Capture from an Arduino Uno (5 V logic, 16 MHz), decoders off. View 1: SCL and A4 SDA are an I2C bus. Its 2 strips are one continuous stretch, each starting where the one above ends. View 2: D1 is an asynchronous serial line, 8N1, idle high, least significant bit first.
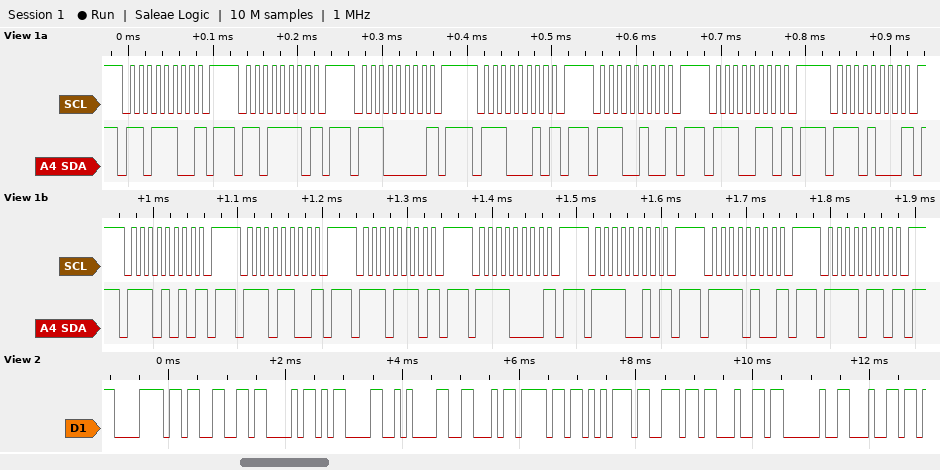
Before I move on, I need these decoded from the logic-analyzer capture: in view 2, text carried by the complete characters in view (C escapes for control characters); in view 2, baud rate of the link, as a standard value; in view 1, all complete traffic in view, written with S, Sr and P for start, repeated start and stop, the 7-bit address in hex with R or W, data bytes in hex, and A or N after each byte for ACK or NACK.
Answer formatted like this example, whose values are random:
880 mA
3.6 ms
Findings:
"x3C\r\nFound d"
9600 baud
S 6EW N P S 6FW N P S 70W N P S 71W N P S 72W N P S 73W N P S 74W N P S 75W N P S 76W N P S 77W N P S 78W N P S 79W N P S 7AW N P S 7BW N P
